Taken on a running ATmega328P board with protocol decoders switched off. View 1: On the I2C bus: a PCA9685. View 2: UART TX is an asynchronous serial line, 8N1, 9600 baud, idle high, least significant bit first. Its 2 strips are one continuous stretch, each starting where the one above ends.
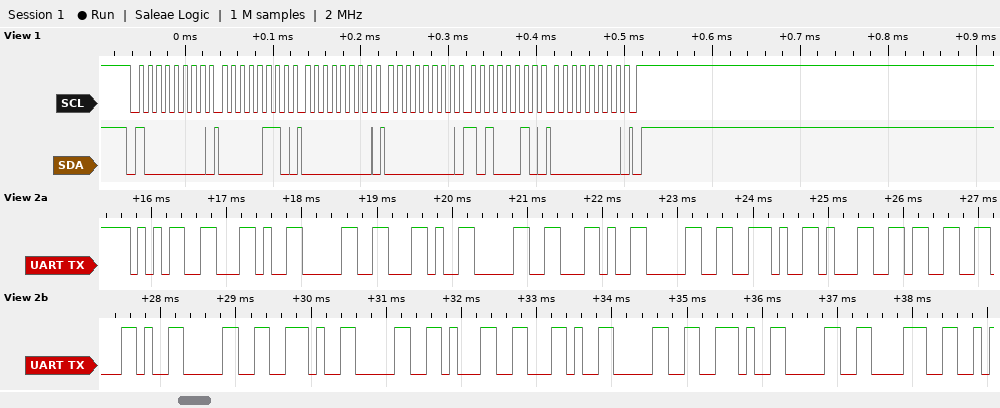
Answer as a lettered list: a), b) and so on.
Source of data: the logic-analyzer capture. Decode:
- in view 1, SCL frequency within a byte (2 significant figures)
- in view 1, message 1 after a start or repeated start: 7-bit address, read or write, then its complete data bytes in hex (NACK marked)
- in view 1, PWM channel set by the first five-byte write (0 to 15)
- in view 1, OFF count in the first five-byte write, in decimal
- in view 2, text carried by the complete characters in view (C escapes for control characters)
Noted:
a) 100 kHz
b) 0x40 write: 06 00 00 A2 00
c) 0
d) 162
e) "5,0,0,0.13,0.01,0.08"
